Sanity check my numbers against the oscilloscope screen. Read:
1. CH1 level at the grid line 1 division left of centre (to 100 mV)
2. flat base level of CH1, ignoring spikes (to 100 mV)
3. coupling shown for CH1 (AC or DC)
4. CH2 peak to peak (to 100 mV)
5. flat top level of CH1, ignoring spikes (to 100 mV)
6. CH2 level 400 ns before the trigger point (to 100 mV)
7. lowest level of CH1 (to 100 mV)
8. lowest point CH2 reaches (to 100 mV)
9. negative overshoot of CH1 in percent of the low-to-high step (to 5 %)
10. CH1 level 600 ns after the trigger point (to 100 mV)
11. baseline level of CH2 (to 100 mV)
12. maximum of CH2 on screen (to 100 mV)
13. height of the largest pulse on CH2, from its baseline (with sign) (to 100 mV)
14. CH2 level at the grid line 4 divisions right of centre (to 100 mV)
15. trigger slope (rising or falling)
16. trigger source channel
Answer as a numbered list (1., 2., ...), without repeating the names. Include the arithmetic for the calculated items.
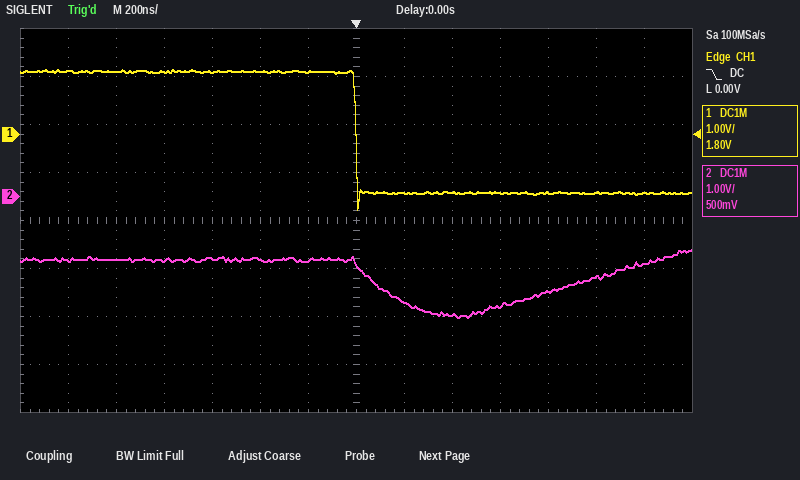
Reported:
1. 1.3 V
2. -1.2 V
3. DC
4. -1.1 V − (-2.5 V) = 1.4 V
5. 1.3 V
6. -1.3 V
7. -1.6 V
8. -2.5 V
9. 15 %
10. -1.2 V
11. -1.3 V
12. -1.1 V
13. -2.5 V − (-1.3 V) = -1.2 V
14. -2.0 V
15. falling
16. CH1
